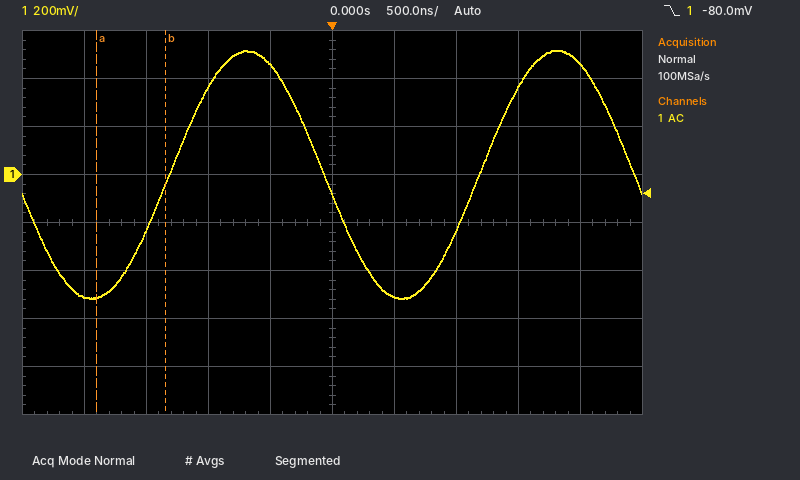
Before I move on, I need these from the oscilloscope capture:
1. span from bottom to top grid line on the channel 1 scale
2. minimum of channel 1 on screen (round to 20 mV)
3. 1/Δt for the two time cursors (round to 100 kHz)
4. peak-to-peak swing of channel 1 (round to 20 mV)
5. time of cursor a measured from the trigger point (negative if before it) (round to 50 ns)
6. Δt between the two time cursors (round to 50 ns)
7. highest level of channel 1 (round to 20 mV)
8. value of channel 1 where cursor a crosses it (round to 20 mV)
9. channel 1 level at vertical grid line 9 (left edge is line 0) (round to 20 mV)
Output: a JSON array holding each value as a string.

["1.6 V", "-520 mV", "1.8 MHz", "1.04 V", "-1.90 µs", "550 ns", "520 mV", "-520 mV", "460 mV"]
